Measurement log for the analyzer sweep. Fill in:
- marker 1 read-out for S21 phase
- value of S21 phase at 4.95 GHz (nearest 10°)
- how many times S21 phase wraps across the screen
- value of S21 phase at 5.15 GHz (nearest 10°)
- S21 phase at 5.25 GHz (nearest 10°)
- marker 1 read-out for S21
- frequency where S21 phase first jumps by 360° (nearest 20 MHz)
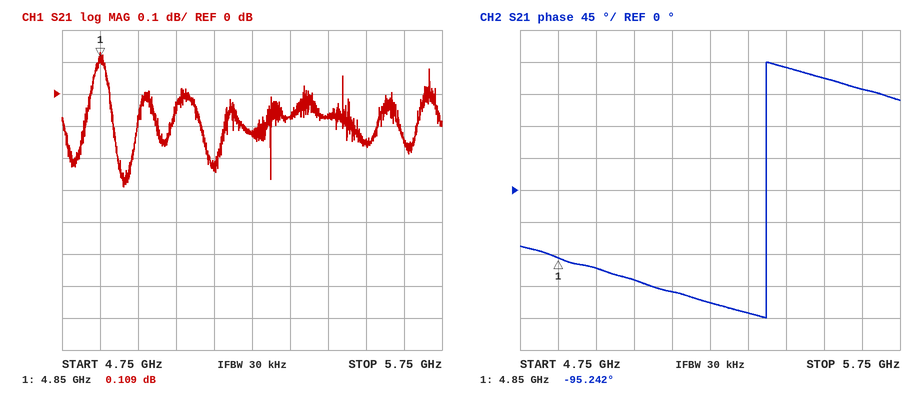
-95.242°
-110°
1
-140°
-160°
0.109 dB
5.40 GHz
